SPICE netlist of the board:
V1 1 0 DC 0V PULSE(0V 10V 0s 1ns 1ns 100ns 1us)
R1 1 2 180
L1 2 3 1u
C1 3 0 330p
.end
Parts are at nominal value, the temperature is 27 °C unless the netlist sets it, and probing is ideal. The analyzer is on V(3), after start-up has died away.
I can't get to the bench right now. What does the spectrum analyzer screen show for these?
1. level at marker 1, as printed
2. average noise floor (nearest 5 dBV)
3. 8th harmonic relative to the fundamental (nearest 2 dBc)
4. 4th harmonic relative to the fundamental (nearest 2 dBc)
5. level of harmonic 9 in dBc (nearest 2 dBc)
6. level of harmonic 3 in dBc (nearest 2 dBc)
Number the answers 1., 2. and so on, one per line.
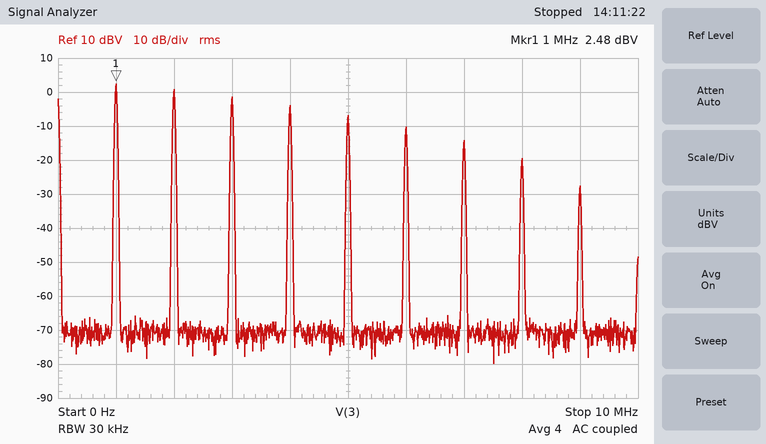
1. 2.48 dBV
2. -70 dBV
3. -22 dBc
4. -6 dBc
5. -30 dBc
6. -4 dBc
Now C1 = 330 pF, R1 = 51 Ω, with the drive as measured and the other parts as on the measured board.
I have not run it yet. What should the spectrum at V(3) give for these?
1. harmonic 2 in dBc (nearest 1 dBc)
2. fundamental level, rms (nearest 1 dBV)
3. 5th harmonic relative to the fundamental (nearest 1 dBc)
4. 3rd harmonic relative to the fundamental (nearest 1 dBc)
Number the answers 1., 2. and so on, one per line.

1. 0 dBc
2. 3 dBV
3. -3 dBc
4. -1 dBc
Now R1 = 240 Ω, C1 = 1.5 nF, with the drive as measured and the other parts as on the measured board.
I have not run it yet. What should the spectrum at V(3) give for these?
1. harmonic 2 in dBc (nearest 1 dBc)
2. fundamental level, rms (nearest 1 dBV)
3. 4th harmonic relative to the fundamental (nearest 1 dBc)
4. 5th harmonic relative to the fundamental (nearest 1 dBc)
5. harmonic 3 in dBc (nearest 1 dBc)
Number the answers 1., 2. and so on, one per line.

1. -6 dBc
2. -5 dBV
3. -14 dBc
4. -17 dBc
5. -10 dBc
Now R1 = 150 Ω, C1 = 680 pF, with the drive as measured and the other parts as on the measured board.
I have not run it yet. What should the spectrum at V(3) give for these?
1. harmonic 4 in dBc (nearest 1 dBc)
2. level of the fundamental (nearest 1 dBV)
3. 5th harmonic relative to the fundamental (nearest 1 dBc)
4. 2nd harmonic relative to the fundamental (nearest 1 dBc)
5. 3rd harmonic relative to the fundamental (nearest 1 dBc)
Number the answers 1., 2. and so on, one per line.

1. -9 dBc
2. 2 dBV
3. -13 dBc
4. -3 dBc
5. -6 dBc
